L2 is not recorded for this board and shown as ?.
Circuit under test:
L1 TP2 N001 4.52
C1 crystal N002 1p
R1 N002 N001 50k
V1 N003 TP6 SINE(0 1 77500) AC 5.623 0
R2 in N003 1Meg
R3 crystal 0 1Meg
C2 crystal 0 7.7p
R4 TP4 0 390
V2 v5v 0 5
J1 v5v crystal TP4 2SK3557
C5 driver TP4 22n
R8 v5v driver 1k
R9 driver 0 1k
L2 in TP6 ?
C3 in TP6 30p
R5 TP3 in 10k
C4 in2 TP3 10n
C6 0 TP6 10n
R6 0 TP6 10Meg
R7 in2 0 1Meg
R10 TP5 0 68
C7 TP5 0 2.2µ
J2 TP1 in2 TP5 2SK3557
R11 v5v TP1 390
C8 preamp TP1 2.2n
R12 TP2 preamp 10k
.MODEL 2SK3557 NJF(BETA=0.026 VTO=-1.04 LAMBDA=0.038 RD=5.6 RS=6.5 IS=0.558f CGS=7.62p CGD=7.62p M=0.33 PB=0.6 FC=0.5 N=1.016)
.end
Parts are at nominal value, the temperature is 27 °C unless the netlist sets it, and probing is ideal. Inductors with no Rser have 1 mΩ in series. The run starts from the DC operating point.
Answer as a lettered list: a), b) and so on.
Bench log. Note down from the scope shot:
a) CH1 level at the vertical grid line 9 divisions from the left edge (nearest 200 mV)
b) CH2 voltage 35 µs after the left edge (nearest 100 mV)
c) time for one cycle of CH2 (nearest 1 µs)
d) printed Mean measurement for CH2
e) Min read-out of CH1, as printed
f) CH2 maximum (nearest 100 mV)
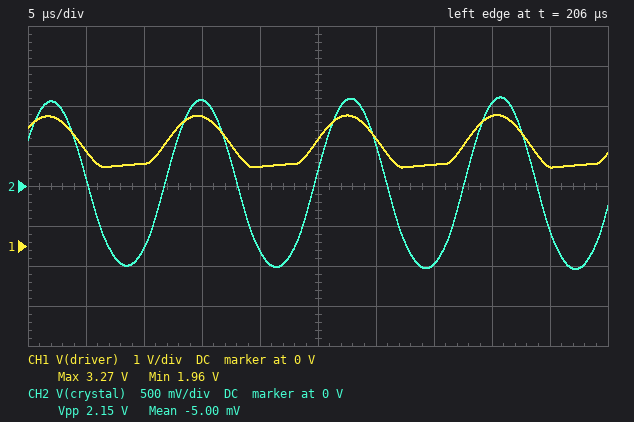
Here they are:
a) 2.0 V
b) -1.0 V
c) 13 µs
d) -5.00 mV
e) 1.96 V
f) 1.1 V
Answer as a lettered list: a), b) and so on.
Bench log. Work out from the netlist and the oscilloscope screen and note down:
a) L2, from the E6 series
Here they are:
a) 100 mH
